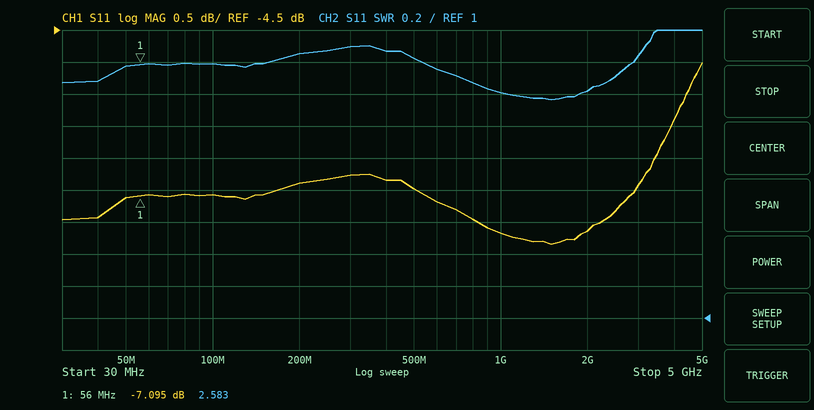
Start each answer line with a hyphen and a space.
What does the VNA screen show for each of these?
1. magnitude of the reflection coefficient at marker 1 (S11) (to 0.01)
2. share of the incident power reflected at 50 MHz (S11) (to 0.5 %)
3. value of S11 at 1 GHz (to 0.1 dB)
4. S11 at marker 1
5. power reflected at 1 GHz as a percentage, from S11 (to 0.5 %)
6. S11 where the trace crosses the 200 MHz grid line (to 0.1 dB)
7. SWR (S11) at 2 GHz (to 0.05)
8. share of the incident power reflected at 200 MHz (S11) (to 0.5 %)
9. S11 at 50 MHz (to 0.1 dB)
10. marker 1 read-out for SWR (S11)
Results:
- 0.44
- 19.5 %
- -7.7 dB
- -7.095 dB
- 17.0 %
- -6.9 dB
- 2.40
- 20.5 %
- -7.1 dB
- 2.583
